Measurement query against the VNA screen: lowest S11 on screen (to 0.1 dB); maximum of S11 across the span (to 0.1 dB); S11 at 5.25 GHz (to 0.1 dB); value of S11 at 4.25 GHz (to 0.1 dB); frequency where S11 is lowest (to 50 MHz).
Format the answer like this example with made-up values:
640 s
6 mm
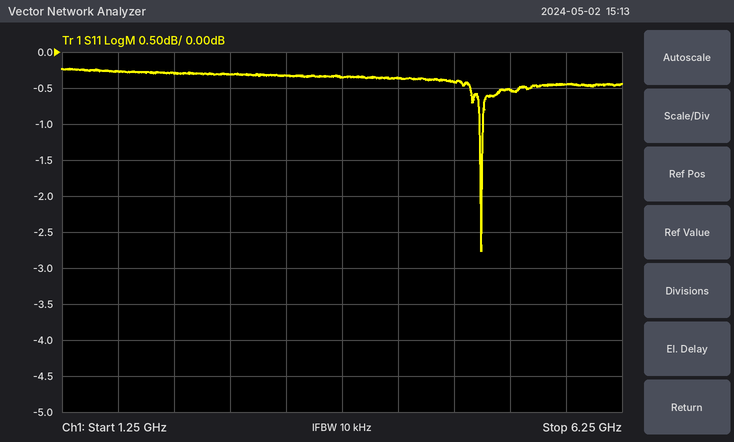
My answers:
-2.8 dB
-0.2 dB
-0.5 dB
-0.4 dB
5.00 GHz
